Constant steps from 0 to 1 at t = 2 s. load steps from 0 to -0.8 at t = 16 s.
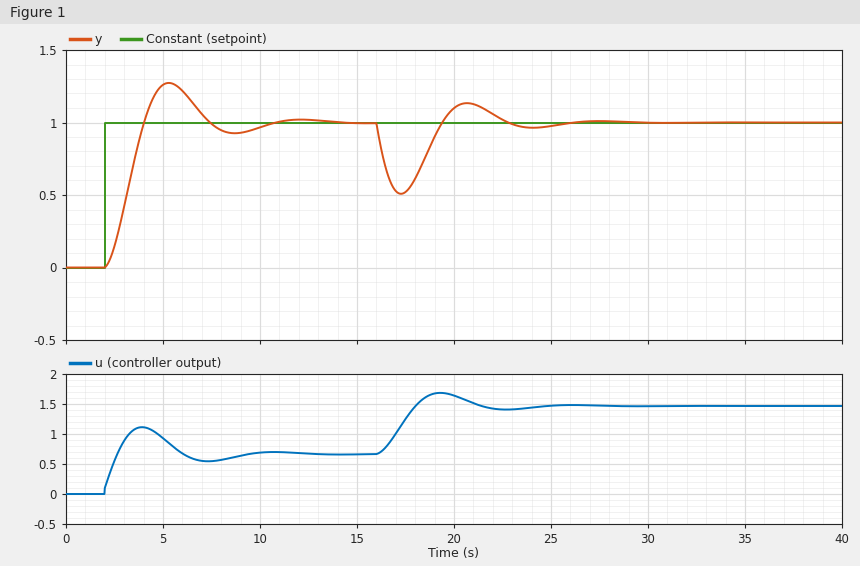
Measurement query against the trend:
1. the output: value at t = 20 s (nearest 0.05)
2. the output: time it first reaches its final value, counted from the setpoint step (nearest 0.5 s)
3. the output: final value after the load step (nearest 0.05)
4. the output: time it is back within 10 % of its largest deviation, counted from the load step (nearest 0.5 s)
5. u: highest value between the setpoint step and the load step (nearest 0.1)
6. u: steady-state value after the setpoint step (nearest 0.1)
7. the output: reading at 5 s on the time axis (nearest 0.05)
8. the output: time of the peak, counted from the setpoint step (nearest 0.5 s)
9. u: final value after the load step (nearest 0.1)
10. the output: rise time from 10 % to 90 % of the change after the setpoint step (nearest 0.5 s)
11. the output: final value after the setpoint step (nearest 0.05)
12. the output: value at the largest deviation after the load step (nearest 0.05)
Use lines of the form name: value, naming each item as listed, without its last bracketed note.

the output: value at t = 20 s: 1.10
the output: time it first reaches its final value, counted from the setpoint step: 2.0 s
the output: final value after the load step: 1.00
the output: time it is back within 10 % of its largest deviation, counted from the load step: 6.0 s
u: highest value between the setpoint step and the load step: 1.1
u: steady-state value after the setpoint step: 0.7
the output: reading at 5 s on the time axis: 1.25
the output: time of the peak, counted from the setpoint step: 3.5 s
u: final value after the load step: 1.5
the output: rise time from 10 % to 90 % of the change after the setpoint step: 1.5 s
the output: final value after the setpoint step: 1.00
the output: value at the largest deviation after the load step: 0.50
